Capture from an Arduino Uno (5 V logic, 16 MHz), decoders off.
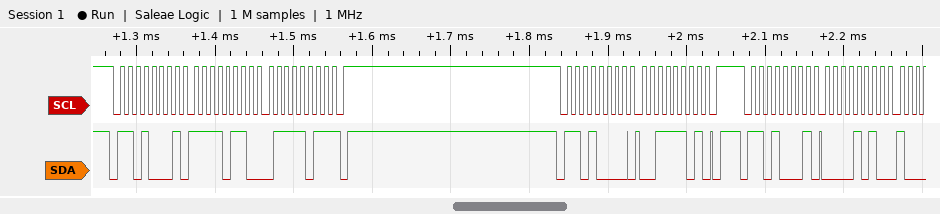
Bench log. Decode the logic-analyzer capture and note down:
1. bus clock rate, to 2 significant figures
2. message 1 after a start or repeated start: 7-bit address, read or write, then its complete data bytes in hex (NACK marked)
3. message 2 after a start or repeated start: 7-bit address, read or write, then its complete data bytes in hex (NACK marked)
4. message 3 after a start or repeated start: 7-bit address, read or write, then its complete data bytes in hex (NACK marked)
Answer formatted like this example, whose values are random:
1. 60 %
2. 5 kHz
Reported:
1. 100 kHz
2. 0x68 read: F6 7B NACK
3. 0x68 write: 3D
4. 0x68 read: 0A
